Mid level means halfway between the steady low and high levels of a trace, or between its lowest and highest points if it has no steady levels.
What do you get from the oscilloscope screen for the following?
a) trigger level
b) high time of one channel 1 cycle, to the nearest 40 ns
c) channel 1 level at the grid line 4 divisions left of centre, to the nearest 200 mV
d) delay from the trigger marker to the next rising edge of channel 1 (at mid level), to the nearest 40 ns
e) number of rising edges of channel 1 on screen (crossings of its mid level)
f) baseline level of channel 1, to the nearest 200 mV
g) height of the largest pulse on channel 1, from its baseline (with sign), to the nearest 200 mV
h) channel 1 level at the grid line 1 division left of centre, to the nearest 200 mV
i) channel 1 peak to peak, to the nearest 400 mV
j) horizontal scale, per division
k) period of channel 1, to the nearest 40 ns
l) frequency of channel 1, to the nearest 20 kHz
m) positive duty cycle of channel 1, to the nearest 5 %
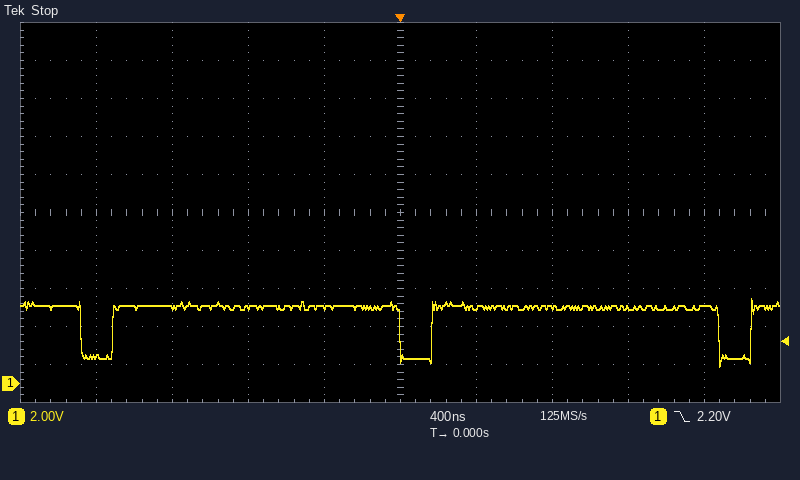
2.20 V
1.52 µs
1.4 V
160 ns
3
4.0 V
-3.2 V
4.0 V
3.6 V
400 ns
1.68 µs
600 kHz
90 %
